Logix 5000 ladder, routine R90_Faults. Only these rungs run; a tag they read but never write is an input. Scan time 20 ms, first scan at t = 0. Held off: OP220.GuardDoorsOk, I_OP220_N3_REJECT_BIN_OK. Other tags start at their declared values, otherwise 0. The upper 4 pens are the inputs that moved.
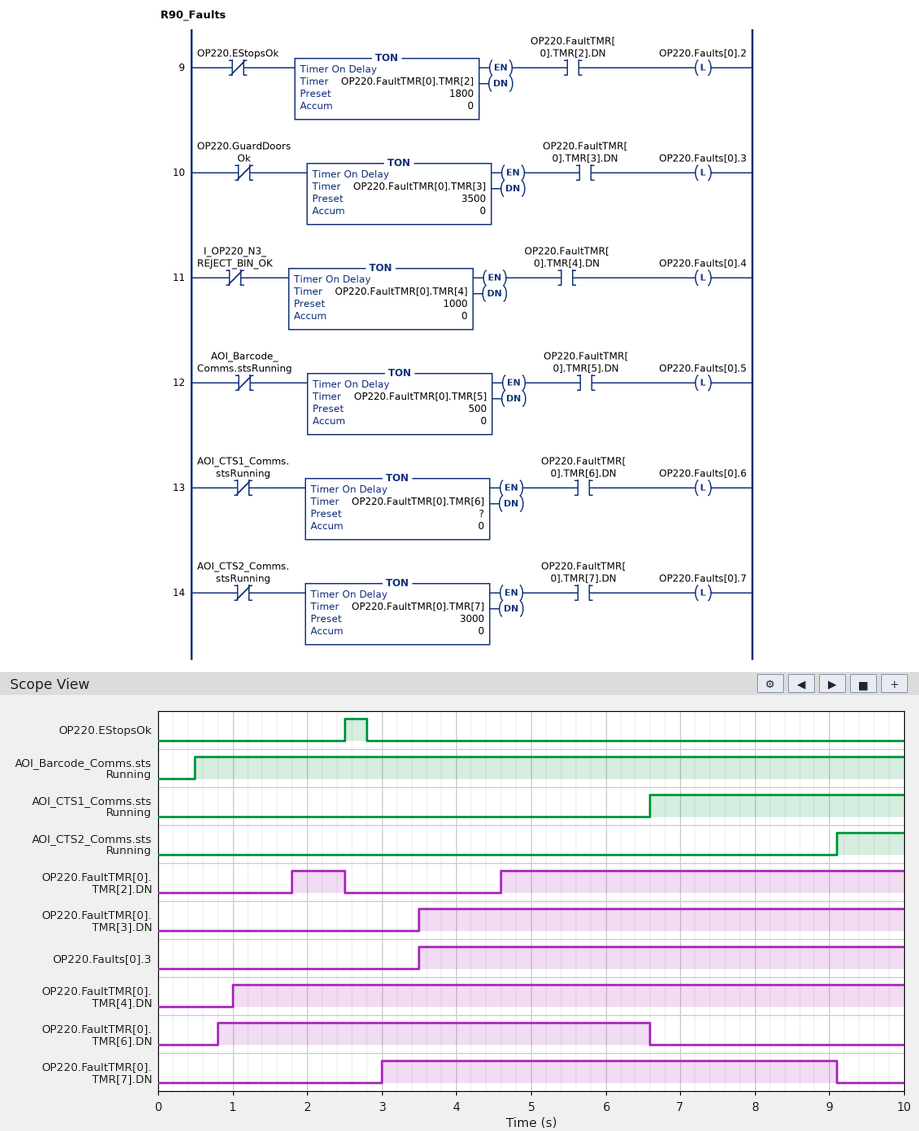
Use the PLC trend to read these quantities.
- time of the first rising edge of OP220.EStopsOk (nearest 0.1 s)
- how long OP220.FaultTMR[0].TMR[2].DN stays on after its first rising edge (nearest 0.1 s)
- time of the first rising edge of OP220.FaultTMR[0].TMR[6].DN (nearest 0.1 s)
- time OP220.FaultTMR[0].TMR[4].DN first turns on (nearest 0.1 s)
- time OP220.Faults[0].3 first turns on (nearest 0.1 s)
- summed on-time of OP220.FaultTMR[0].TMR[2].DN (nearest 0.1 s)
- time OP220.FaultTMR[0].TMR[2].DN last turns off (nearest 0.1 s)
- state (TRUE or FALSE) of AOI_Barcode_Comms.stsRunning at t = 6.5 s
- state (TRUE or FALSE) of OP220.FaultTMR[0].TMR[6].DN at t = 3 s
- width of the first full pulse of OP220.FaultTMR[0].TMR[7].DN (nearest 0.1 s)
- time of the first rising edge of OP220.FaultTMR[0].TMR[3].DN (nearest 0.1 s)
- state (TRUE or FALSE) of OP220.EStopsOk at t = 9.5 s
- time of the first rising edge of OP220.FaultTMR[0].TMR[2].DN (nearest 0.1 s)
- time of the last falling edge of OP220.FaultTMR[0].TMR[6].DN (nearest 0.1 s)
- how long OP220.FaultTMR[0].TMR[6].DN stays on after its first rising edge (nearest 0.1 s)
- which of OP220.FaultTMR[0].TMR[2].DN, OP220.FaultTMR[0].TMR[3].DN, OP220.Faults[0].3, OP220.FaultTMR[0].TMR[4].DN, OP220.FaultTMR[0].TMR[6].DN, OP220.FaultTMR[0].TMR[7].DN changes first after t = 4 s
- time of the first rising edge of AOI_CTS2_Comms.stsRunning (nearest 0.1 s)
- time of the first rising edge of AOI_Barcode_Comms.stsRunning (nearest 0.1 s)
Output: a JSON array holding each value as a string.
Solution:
["2.5 s", "0.7 s", "0.8 s", "1.0 s", "3.5 s", "6.1 s", "2.5 s", "TRUE", "TRUE", "6.1 s", "3.5 s", "FALSE", "1.8 s", "6.6 s", "5.8 s", "OP220.FaultTMR[0].TMR[2].DN", "9.1 s", "0.5 s"]
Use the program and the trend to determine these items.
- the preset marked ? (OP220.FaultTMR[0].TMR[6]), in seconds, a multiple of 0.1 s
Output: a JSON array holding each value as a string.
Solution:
["0.8 s"]
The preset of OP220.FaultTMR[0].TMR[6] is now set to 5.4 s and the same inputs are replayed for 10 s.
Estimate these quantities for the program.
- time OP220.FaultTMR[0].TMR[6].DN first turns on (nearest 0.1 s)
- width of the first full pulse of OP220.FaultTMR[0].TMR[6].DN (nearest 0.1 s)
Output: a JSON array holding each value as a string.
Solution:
["5.4 s", "1.2 s"]
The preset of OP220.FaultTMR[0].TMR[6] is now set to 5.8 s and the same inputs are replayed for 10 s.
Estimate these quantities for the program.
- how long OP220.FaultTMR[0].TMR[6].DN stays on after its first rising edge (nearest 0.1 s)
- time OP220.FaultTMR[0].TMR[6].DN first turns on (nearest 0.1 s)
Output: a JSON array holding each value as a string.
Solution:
["0.8 s", "5.8 s"]
